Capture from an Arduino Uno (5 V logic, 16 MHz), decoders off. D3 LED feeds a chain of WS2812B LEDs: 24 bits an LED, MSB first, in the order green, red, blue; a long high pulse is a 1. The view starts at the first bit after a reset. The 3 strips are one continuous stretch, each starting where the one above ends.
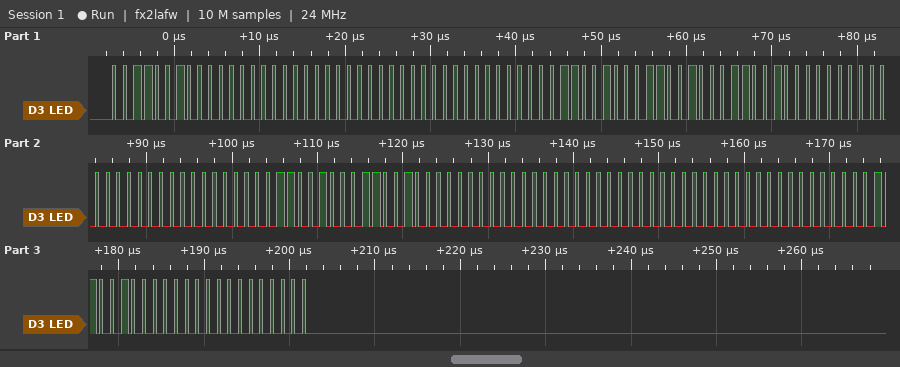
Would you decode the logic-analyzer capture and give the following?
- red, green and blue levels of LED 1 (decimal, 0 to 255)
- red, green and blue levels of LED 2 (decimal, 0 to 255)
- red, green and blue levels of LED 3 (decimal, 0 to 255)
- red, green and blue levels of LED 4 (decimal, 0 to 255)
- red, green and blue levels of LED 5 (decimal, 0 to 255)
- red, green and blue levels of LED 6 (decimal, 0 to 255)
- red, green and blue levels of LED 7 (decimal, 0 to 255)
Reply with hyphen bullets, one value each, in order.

- 0, 50, 0
- 0, 0, 50
- 50, 50, 0
- 0, 0, 50
- 0, 50, 0
- 0, 0, 0
- 0, 50, 0
